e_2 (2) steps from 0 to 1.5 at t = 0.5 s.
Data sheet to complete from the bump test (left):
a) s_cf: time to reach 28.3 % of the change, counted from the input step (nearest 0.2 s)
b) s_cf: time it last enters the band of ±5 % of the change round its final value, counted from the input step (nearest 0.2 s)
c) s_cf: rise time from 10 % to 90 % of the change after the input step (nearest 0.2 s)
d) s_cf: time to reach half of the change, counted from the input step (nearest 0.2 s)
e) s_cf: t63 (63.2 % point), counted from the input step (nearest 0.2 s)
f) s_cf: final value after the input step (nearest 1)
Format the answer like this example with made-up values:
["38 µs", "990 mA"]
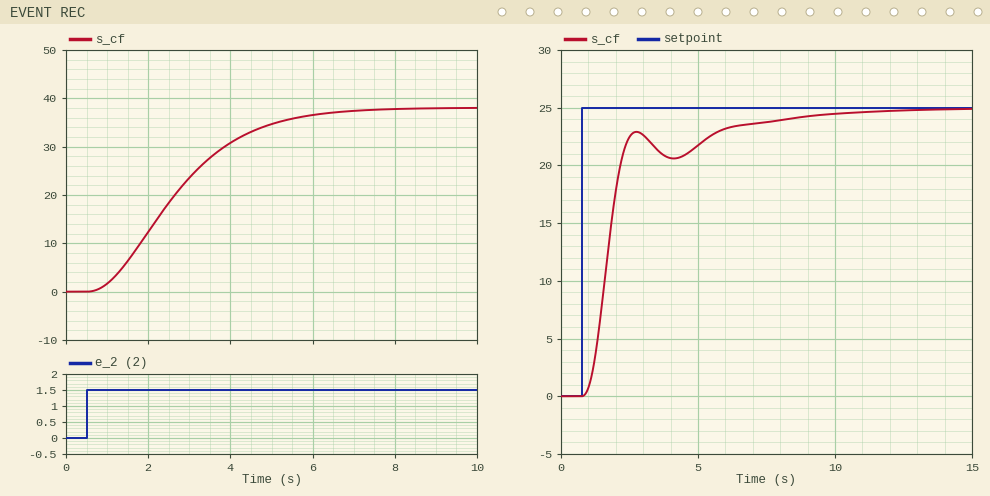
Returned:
["1.4 s", "5.2 s", "3.6 s", "2.0 s", "2.6 s", "38"]
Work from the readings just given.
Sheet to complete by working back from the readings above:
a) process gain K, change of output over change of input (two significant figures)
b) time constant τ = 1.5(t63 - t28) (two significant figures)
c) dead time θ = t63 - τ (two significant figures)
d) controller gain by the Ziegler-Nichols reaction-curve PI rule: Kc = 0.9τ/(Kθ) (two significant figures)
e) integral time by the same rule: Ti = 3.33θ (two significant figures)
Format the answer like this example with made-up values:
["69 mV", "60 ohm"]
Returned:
["25", "1.8 s", "0.80 s", "0.081", "2.7 s"]
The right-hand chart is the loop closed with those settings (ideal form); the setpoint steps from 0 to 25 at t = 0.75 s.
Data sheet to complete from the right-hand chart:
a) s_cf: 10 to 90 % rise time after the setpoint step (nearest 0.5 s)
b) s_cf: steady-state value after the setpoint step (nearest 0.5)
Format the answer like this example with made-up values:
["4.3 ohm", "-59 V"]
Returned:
["1.5 s", "25.0"]
